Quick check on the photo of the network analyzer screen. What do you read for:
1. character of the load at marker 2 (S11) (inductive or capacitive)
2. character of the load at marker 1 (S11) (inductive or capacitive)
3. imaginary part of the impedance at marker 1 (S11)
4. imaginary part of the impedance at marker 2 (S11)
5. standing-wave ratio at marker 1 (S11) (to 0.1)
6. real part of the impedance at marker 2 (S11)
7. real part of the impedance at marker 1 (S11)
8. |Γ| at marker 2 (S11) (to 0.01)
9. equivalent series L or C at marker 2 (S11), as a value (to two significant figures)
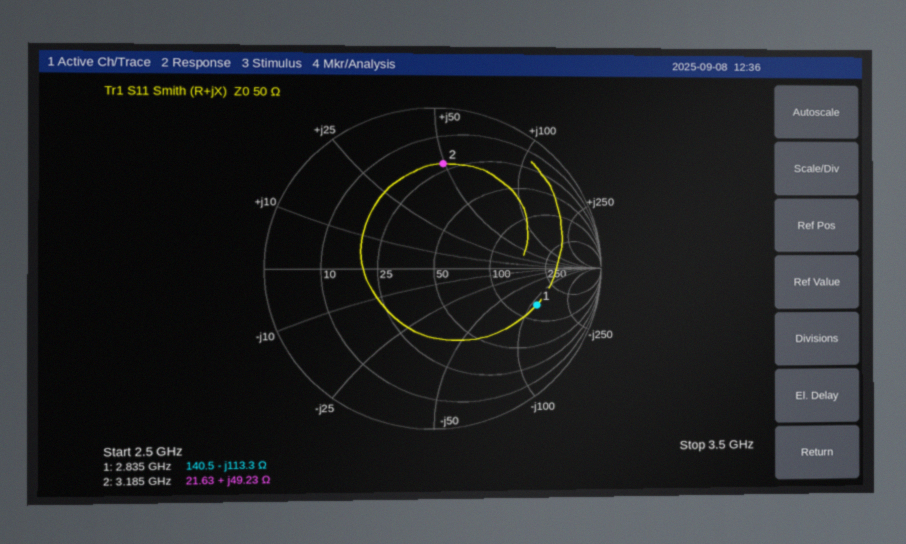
inductive
capacitive
-113.3 Ω
+49.23 Ω
4.8
21.63 Ω
140.5 Ω
0.65
2.5 nH
